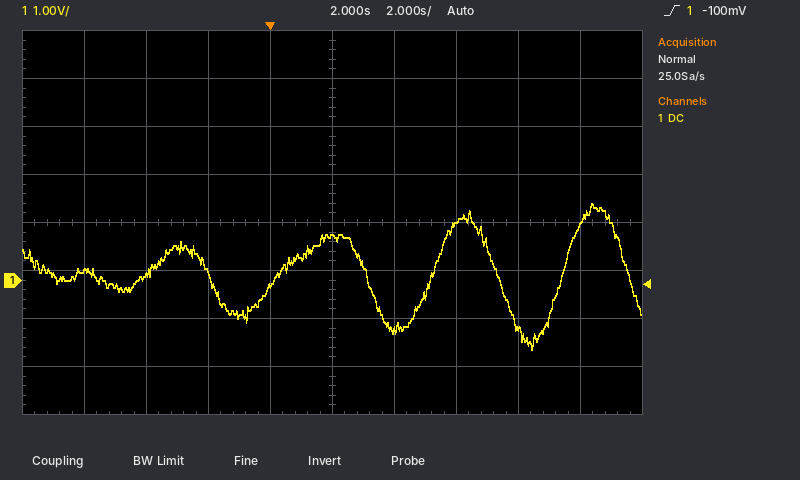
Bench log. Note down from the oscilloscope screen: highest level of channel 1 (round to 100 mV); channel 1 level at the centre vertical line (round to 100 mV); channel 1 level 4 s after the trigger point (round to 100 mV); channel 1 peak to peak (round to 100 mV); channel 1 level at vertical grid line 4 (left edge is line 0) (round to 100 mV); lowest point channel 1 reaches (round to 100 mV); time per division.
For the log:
1.6 V
900 mV
-1.0 V
3.0 V
-100 mV
-1.4 V
2 s
